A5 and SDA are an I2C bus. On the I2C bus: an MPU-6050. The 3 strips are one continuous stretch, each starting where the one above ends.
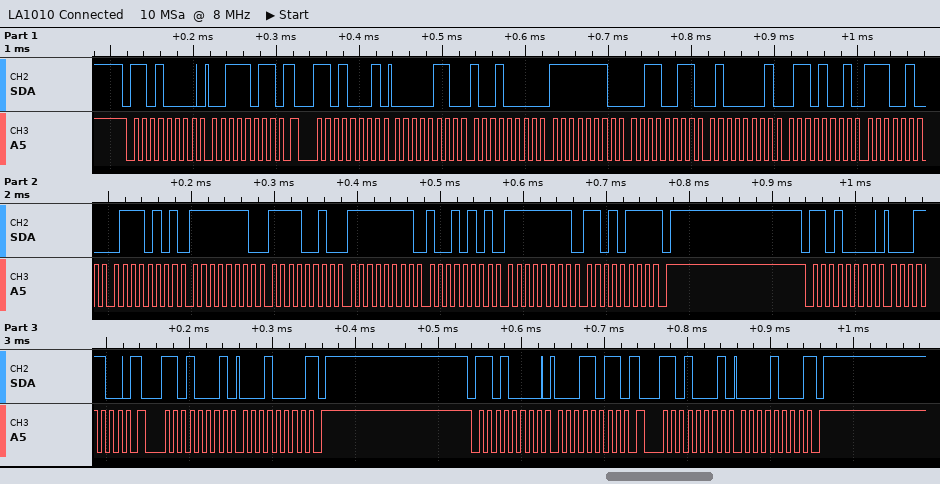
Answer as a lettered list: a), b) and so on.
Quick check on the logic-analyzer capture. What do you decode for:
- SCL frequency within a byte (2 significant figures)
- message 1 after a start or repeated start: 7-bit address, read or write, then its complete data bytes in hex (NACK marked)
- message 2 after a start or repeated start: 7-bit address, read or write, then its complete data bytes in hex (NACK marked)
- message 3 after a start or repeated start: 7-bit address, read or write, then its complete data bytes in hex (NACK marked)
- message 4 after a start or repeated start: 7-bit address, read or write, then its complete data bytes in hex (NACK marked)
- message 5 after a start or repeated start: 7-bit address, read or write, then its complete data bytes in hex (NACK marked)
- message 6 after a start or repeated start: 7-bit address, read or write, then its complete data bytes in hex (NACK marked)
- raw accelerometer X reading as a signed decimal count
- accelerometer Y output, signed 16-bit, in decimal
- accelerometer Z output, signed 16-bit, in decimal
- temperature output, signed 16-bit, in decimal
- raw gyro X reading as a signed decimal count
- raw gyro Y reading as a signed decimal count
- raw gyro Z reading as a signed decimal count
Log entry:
a) 100 kHz
b) 0x68 write: 3B
c) 0x68 read: 06 90 FE 33 41 69 E4 75 FE F2 FF 95 FF D7 NACK
d) 0x68 write: 1C
e) 0x68 read: 10 NACK
f) 0x68 write: 1B
g) 0x68 read: 08 NACK
h) 1680
i) -461
j) 16745
k) -7051
l) -270
m) -107
n) -41
